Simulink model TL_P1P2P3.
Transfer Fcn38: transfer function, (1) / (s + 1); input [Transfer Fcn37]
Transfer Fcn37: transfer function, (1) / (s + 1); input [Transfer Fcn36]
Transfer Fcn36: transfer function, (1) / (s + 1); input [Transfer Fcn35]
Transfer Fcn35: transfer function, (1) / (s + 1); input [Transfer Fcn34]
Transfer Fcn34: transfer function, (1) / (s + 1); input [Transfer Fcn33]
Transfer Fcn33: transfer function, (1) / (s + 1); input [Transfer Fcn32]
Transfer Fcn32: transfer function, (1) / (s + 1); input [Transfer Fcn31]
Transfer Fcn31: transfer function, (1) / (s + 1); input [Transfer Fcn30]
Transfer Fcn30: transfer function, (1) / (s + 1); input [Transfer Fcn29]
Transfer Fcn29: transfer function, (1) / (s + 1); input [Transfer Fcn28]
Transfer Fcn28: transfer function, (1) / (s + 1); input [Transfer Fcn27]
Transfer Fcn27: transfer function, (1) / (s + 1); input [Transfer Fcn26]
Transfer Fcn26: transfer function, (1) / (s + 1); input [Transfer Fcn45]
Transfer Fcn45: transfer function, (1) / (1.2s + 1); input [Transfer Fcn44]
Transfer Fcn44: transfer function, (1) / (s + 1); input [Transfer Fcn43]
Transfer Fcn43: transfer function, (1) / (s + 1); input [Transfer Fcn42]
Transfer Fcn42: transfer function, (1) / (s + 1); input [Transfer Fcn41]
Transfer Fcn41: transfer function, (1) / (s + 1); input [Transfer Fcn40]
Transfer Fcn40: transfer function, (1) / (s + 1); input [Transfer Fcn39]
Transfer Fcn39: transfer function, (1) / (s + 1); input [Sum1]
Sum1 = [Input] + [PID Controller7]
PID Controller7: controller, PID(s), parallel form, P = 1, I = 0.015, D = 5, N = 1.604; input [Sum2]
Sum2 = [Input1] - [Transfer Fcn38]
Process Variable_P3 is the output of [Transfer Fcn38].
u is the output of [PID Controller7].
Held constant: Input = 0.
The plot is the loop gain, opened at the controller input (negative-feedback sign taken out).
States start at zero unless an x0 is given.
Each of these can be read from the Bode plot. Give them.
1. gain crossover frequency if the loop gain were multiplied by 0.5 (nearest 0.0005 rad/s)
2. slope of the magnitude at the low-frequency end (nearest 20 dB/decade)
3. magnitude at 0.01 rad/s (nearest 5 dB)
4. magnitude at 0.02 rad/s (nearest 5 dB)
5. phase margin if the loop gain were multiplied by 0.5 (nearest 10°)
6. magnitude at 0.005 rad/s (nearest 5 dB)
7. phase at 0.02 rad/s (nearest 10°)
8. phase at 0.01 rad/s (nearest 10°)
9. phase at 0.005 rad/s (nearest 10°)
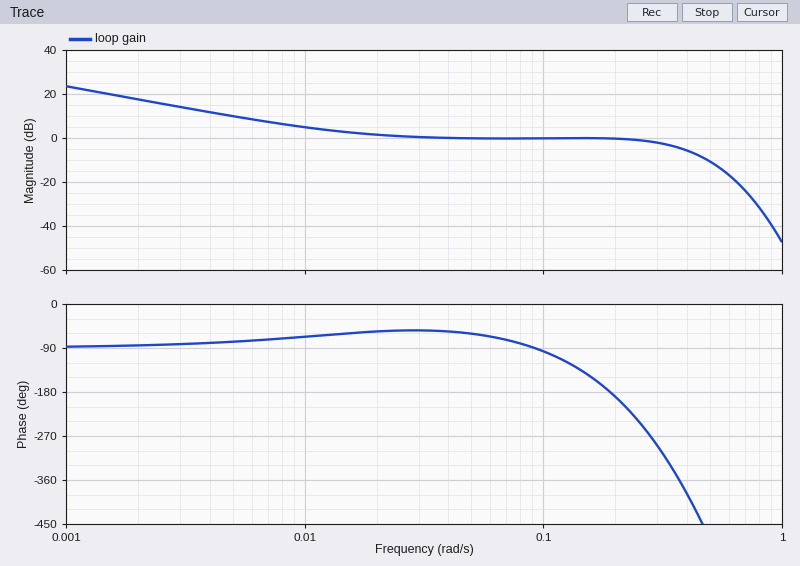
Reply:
0.0085 rad/s
-20 dB/decade
5 dB
0 dB
110°
10 dB
-60°
-70°
-80°
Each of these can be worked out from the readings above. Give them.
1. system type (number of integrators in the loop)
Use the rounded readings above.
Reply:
1
